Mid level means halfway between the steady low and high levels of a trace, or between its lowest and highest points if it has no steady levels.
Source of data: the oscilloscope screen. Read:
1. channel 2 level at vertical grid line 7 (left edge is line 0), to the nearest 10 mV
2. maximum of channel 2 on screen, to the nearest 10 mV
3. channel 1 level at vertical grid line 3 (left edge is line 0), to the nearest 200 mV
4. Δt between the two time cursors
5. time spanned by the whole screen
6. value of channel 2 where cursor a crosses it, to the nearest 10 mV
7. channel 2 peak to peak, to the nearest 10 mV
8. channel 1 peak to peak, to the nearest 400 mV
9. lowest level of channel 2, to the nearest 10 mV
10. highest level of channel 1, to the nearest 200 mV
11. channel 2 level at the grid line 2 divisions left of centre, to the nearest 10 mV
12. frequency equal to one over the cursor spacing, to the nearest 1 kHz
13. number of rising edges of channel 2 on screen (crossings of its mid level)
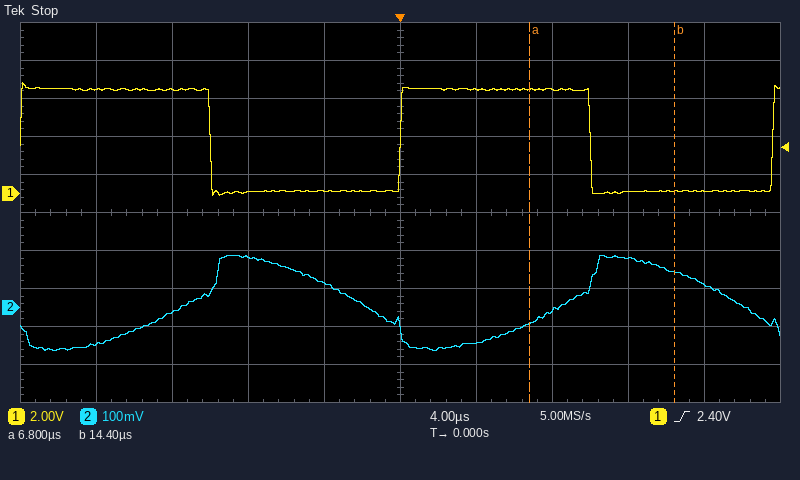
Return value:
-10 mV
140 mV
0.0 V
7.6 µs
40 µs
-40 mV
250 mV
6.0 V
-110 mV
5.8 V
130 mV
132 kHz
2
